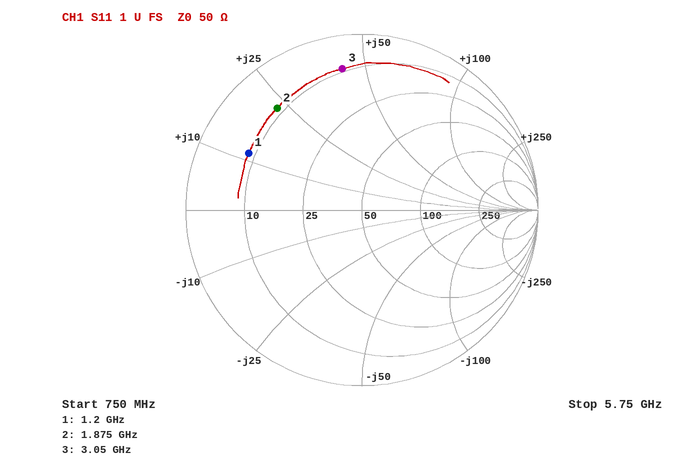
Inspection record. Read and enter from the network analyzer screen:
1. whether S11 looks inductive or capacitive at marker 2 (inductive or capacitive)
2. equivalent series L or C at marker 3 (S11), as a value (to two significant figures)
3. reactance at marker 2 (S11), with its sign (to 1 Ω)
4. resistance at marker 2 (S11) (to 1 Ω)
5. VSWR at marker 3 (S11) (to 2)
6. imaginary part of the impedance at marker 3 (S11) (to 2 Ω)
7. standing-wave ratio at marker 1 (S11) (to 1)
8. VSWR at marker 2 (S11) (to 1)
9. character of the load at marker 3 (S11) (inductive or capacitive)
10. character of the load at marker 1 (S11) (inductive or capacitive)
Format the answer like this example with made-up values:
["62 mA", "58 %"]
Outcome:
["inductive", "2.2 nH", "+23 Ω", "9 Ω", "10", "+42 Ω", "6", "7", "inductive", "inductive"]
